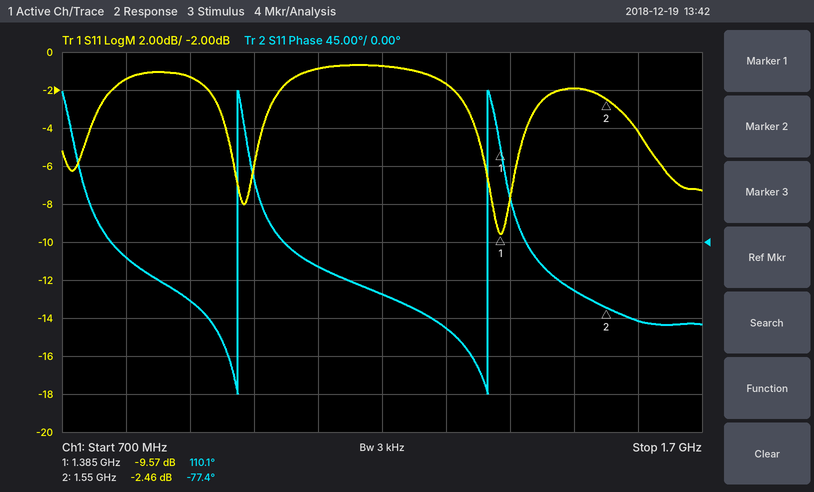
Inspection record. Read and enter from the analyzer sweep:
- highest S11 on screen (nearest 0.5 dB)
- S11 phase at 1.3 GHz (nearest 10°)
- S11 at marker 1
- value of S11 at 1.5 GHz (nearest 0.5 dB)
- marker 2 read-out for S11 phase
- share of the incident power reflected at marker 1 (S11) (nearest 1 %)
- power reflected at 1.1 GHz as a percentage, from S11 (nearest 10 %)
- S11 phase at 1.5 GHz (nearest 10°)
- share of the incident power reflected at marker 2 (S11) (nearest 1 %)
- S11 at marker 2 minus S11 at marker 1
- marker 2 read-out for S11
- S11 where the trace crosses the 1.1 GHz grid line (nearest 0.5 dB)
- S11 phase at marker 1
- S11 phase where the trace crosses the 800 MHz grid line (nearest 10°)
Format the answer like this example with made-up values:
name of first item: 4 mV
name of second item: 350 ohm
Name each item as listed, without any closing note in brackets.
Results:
highest S11 on screen: -0.5 dB
S11 phase at 1.3 GHz: -100°
S11 at marker 1: -9.57 dB
value of S11 at 1.5 GHz: -2.0 dB
marker 2 read-out for S11 phase: -77.4°
share of the incident power reflected at marker 1 (S11): 11 %
power reflected at 1.1 GHz as a percentage, from S11: 80 %
S11 phase at 1.5 GHz: -60°
share of the incident power reflected at marker 2 (S11): 57 %
S11 at marker 2 minus S11 at marker 1: 7.11 dB
marker 2 read-out for S11: -2.46 dB
S11 where the trace crosses the 1.1 GHz grid line: -1.0 dB
S11 phase at marker 1: 110.1°
S11 phase where the trace crosses the 800 MHz grid line: -20°
